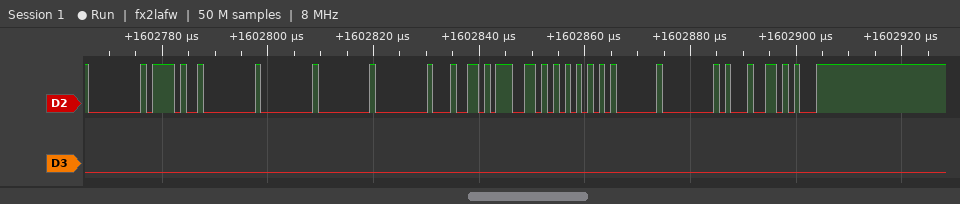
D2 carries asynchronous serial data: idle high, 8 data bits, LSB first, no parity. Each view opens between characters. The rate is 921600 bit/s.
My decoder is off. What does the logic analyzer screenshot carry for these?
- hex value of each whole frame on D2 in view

00, 2F, 00, 00, 00, 00, 64, 67, 55, 01, 00, 91, C5
